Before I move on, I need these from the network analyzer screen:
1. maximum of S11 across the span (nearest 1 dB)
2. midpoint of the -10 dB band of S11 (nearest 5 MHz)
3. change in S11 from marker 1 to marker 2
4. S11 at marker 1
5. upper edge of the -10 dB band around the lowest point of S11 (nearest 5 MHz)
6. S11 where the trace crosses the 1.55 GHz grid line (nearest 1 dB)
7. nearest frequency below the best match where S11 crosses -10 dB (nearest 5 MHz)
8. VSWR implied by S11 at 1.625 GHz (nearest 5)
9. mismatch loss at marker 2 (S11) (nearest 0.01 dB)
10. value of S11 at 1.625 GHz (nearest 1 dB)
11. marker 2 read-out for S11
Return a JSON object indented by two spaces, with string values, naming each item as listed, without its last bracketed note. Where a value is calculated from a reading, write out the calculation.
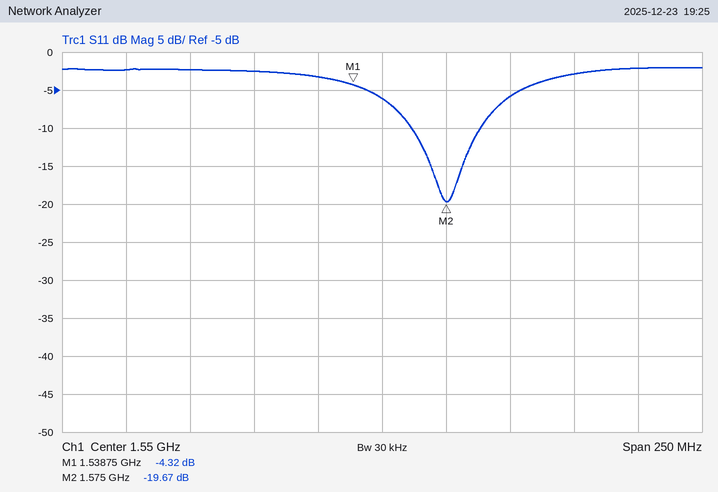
{
  "maximum of S11 across the span": "-2 dB",
  "midpoint of the -10 dB band of S11": "1.575 GHz",
  "change in S11 from marker 1 to marker 2": "-19.67 − (-4.32) = -15.35 dB",
  "S11 at marker 1": "-4.32 dB",
  "upper edge of the -10 dB band around the lowest point of S11": "1.590 GHz",
  "S11 where the trace crosses the 1.55 GHz grid line": "-6 dB",
  "nearest frequency below the best match where S11 crosses -10 dB": "1.560 GHz",
  "VSWR implied by S11 at 1.625 GHz": "|Γ| = 10^(-3/20) = 0.7079; VSWR = (1 + 0.7079)/(1 − 0.7079) ≈ 5.85, so 5 to the nearest 5",
  "mismatch loss at marker 2 (S11)": "−10 log10(1 − 10^(-19.67/10)) ≈ 0.05 dB",
  "value of S11 at 1.625 GHz": "-3 dB",
  "marker 2 read-out for S11": "-19.67 dB"
}
